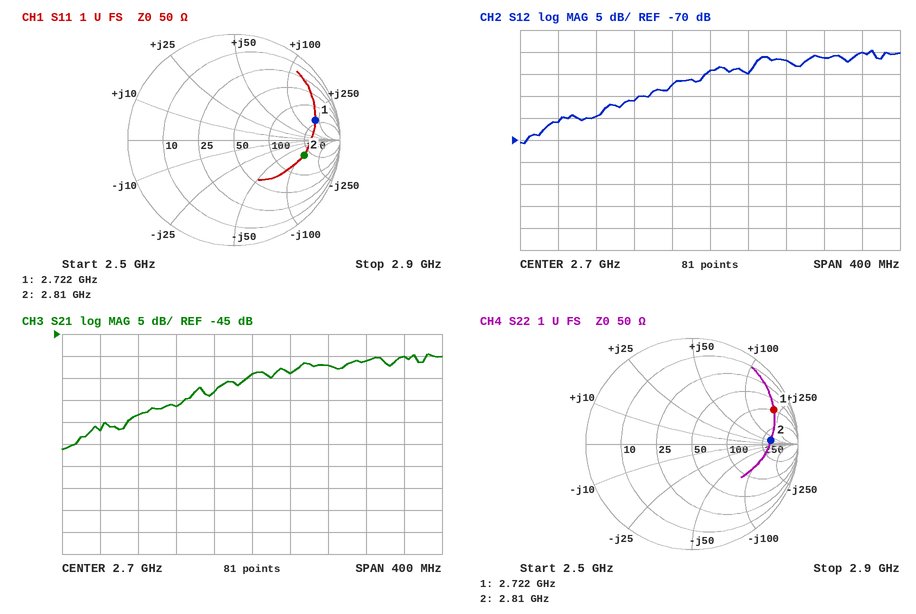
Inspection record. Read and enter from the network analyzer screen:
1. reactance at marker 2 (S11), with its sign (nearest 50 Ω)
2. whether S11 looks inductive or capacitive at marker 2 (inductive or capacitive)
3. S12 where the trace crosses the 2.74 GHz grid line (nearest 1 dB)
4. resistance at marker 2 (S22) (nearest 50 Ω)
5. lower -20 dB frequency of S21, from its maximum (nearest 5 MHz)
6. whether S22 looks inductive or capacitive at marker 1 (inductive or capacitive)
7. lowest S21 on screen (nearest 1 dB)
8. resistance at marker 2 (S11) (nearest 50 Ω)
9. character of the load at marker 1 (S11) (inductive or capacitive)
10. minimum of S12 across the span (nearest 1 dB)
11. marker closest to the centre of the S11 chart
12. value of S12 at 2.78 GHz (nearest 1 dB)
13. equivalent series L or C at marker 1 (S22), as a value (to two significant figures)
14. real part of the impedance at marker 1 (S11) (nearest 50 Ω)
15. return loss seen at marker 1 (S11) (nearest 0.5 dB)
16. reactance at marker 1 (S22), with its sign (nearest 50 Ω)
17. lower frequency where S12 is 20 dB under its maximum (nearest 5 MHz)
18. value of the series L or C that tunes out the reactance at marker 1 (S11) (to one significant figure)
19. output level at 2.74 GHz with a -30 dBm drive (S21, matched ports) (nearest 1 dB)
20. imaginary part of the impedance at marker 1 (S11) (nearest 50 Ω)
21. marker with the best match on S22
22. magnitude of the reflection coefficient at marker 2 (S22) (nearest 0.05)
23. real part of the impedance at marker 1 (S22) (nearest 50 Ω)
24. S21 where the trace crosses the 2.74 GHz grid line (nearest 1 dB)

-100 Ω
capacitive
-55 dB
350 Ω
2.515 GHz
inductive
-71 dB
200 Ω
inductive
-71 dB
marker 2
-52 dB
12 nH
200 Ω
2.0 dB
+200 Ω
2.510 GHz
300 fF
-84 dBm
+200 Ω
marker 2
0.75
100 Ω
-54 dB
